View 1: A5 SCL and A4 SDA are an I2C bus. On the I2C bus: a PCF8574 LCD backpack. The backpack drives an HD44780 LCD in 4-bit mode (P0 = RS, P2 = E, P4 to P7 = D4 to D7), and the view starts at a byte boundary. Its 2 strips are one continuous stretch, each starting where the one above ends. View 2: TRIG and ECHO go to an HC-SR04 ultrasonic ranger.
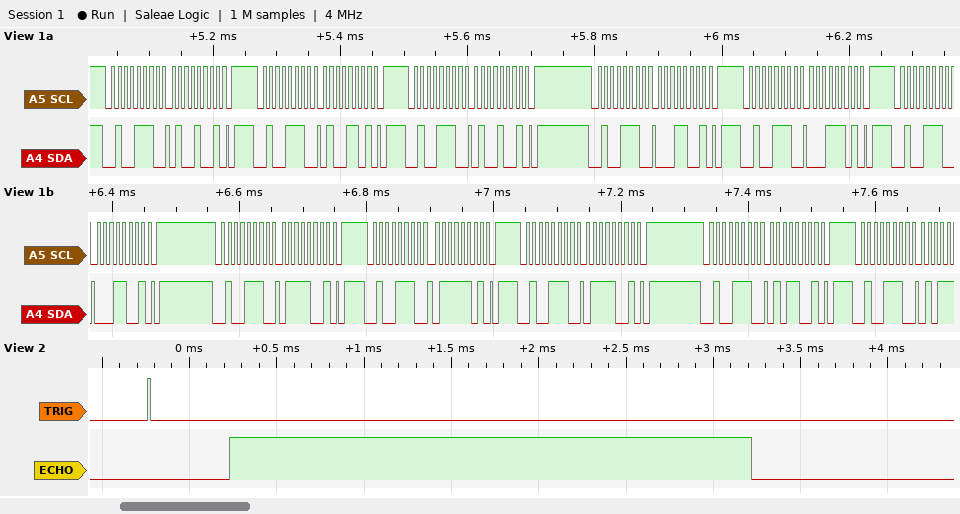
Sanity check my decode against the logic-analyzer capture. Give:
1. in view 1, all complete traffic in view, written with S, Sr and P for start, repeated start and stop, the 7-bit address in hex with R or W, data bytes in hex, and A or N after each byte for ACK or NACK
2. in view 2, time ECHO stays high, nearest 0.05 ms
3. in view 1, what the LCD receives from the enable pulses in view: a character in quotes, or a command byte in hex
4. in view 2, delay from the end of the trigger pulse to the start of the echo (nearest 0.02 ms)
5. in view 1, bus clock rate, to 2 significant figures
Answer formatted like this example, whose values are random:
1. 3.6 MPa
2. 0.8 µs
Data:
1. S 27W A 49 A P S 27W A 4D A P S 27W A 49 A P S 27W A 19 A P S 27W A 1D A P S 27W A 19 A P S 27W A 79 A P S 27W A 7D A P S 27W A 79 A P S 27W A 59 A P S 27W A
2. 3.00 ms
3. 'A'
4. 0.46 ms
5. 100 kHz
